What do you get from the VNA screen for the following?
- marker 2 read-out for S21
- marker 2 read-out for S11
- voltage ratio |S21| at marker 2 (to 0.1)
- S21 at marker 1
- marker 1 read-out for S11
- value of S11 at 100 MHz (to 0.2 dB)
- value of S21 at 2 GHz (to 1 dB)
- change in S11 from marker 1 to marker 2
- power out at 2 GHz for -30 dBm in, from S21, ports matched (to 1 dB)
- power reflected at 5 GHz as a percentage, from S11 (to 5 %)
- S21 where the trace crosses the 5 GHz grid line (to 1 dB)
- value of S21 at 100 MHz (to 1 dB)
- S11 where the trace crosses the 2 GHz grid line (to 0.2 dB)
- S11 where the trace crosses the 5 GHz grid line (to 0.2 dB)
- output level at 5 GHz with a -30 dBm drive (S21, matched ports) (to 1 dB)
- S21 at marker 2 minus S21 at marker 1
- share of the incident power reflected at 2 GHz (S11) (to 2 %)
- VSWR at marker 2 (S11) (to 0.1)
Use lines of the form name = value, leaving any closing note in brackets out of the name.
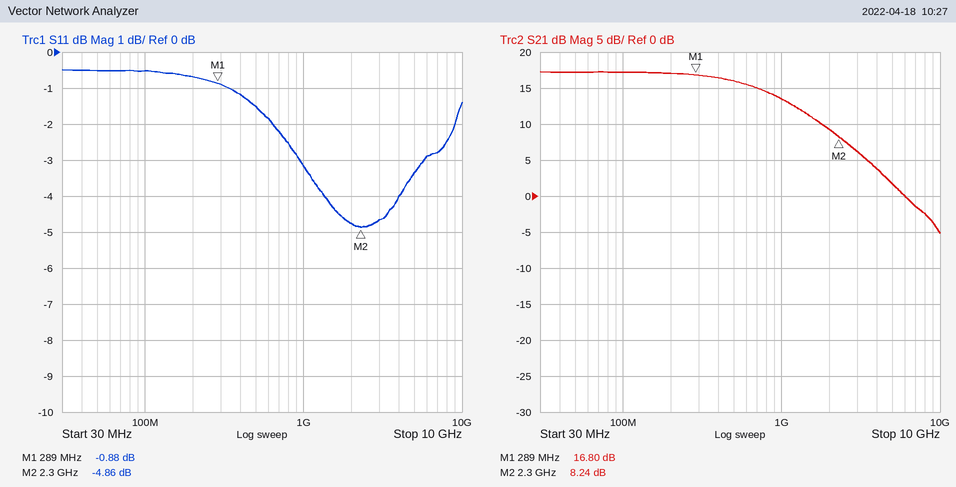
marker 2 read-out for S21 = 8.24 dB
marker 2 read-out for S11 = -4.86 dB
voltage ratio |S21| at marker 2 = 2.6
S21 at marker 1 = 16.80 dB
marker 1 read-out for S11 = -0.88 dB
value of S11 at 100 MHz = -0.6 dB
value of S21 at 2 GHz = 9 dB
change in S11 from marker 1 to marker 2 = -3.98 dB
power out at 2 GHz for -30 dBm in, from S21, ports matched = -21 dBm
power reflected at 5 GHz as a percentage, from S11 = 45 %
S21 where the trace crosses the 5 GHz grid line = 2 dB
value of S21 at 100 MHz = 17 dB
S11 where the trace crosses the 2 GHz grid line = -4.8 dB
S11 where the trace crosses the 5 GHz grid line = -3.4 dB
output level at 5 GHz with a -30 dBm drive (S21, matched ports) = -28 dBm
S21 at marker 2 minus S21 at marker 1 = -8.56 dB
share of the incident power reflected at 2 GHz (S11) = 34 %
VSWR at marker 2 (S11) = 3.7
